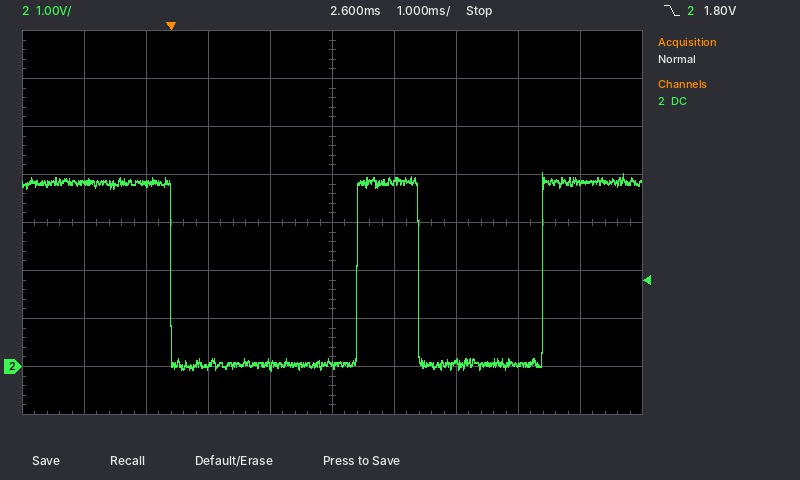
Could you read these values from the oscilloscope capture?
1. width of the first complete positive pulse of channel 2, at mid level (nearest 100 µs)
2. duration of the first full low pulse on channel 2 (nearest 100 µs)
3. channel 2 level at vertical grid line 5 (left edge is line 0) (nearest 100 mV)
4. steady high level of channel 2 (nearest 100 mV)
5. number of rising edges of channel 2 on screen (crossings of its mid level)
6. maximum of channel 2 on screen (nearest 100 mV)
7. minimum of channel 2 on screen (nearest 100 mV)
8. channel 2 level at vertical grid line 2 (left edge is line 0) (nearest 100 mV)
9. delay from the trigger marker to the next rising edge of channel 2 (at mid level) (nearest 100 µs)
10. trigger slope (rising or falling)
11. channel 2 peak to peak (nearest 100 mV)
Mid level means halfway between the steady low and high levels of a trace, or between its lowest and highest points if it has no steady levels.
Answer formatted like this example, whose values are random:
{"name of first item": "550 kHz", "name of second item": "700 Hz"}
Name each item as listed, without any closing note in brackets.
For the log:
{"width of the first complete positive pulse of channel 2, at mid level": "1.0 ms", "duration of the first full low pulse on channel 2": "3.0 ms", "channel 2 level at vertical grid line 5 (left edge is line 0)": "0.0 V", "steady high level of channel 2": "3.8 V", "number of rising edges of channel 2 on screen": "2", "maximum of channel 2 on screen": "4.0 V", "minimum of channel 2 on screen": "-100 mV", "channel 2 level at vertical grid line 2 (left edge is line 0)": "3.8 V", "delay from the trigger marker to the next rising edge of channel 2 (at mid level)": "3.0 ms", "trigger slope": "falling", "channel 2 peak to peak": "4.1 V"}
